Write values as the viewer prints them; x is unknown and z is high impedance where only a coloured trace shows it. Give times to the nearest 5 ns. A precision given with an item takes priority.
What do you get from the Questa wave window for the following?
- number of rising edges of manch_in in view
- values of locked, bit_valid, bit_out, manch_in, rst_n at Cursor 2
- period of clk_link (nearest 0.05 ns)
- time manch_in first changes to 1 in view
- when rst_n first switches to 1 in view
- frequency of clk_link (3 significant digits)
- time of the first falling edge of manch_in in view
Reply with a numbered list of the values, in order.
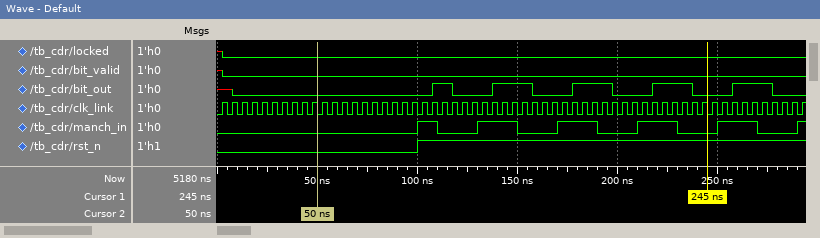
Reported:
1. 6
2. locked=0, bit_valid=0, bit_out=0, manch_in=0, rst_n=0
3. 5 ns
4. 100 ns
5. 100 ns
6. 200 MHz
7. 110 ns
